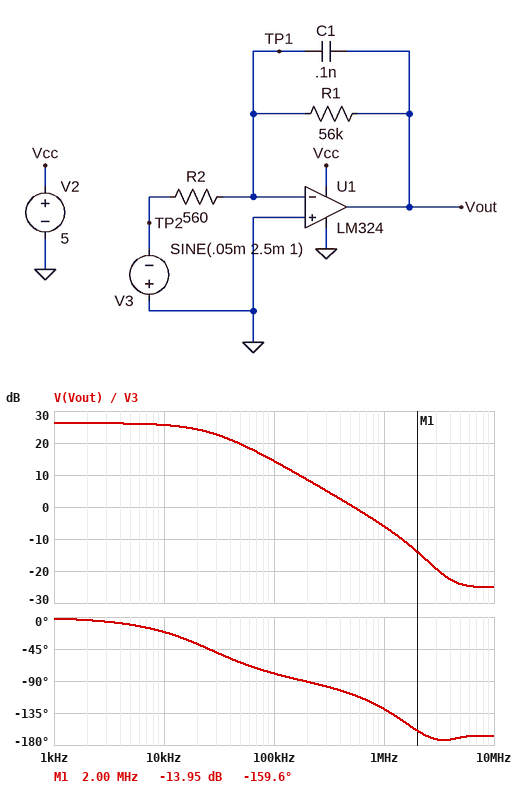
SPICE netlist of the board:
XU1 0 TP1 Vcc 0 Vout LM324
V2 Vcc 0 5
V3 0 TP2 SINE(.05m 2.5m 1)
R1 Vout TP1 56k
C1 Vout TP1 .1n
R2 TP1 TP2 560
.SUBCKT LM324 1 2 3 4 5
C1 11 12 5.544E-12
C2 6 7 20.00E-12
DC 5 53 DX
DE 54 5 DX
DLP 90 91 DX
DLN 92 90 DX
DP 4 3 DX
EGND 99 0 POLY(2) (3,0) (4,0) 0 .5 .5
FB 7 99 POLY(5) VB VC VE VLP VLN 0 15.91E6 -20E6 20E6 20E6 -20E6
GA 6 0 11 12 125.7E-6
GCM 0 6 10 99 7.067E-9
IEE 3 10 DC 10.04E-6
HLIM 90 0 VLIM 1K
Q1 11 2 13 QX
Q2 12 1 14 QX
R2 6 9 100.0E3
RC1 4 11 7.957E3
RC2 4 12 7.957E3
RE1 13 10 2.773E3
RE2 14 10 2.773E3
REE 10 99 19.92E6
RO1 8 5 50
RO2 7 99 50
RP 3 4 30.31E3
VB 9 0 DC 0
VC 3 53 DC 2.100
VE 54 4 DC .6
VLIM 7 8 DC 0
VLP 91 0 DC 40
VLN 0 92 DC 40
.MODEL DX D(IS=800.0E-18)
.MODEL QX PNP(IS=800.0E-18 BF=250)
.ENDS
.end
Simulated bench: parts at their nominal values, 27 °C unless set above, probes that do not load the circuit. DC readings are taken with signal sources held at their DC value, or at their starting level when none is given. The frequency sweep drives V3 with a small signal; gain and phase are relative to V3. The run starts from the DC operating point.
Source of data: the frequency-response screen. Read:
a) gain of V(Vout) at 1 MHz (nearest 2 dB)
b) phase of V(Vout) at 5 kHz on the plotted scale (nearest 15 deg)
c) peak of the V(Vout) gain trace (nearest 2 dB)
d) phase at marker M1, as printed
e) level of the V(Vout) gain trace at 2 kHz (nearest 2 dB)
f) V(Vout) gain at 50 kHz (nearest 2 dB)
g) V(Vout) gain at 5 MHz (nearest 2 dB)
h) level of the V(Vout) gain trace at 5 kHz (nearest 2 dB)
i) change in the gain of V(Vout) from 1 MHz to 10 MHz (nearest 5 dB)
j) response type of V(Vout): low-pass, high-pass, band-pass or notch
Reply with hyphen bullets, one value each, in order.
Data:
- -6 dB
- -15 deg
- 26 dB
- -159.6 deg
- 26 dB
- 20 dB
- -24 dB
- 26 dB
- -20 dB
- low-pass
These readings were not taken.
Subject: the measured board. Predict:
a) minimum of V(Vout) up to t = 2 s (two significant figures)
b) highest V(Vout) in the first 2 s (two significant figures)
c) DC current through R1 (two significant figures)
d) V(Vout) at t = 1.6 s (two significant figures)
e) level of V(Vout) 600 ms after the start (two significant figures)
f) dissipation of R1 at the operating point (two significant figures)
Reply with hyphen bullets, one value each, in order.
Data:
- 88 mV
- 270 mV
- 2.1 µA
- 97 mV
- 97 mV
- 240 nW
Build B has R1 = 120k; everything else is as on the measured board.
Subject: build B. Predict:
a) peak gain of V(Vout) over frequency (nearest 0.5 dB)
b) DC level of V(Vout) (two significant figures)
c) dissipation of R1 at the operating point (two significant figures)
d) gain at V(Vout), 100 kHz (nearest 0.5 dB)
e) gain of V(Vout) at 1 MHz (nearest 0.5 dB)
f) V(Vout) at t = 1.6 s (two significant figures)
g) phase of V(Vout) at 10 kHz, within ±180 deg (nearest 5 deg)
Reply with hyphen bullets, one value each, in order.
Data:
- 33.0 dB
- 140 mV
- 160 nW
- 16.0 dB
- -4.5 dB
- 100 mV
- -35 deg
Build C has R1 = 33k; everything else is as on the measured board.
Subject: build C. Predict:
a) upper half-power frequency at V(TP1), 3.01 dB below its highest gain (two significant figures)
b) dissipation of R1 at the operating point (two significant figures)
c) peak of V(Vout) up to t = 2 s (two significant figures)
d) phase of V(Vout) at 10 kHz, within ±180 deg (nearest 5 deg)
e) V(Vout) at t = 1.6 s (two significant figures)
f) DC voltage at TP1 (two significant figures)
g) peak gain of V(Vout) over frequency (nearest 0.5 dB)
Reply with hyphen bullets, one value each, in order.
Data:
- 3.8 MHz
- 330 nW
- 170 mV
- -15 deg
- 91 mV
- 1.7 mV
- 22.0 dB
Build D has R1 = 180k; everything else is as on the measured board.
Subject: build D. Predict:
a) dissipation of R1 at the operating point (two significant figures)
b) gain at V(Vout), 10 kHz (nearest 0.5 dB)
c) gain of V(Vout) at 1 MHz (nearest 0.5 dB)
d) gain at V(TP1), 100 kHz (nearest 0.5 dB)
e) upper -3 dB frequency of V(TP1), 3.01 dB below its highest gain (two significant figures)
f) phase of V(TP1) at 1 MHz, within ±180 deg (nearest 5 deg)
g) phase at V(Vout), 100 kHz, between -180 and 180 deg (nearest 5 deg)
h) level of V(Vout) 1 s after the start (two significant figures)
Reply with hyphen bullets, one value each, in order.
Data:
- 120 nW
- 33.5 dB
- -4.0 dB
- -2.5 dB
- 4.1 MHz
- 170 deg
- -90 deg
- 150 mV
